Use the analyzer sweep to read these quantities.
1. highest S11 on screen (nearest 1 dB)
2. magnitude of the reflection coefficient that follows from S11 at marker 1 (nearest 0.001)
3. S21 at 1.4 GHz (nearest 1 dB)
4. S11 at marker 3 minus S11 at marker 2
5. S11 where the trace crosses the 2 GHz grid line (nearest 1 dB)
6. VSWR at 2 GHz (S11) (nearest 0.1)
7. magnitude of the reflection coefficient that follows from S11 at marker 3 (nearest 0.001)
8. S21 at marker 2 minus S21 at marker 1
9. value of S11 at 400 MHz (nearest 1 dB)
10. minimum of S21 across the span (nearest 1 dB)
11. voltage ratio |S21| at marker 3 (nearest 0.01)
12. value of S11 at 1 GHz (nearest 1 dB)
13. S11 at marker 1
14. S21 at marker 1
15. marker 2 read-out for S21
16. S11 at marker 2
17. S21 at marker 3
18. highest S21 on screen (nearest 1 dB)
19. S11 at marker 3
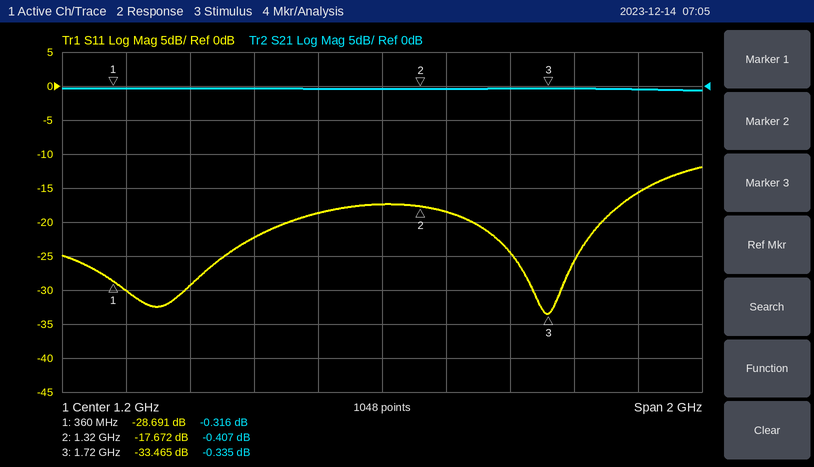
-12 dB
0.037
0 dB
-15.793 dB
-16 dB
1.4
0.021
-0.091 dB
-30 dB
-1 dB
0.96
-19 dB
-28.691 dB
-0.316 dB
-0.407 dB
-17.672 dB
-0.335 dB
0 dB
-33.465 dB
